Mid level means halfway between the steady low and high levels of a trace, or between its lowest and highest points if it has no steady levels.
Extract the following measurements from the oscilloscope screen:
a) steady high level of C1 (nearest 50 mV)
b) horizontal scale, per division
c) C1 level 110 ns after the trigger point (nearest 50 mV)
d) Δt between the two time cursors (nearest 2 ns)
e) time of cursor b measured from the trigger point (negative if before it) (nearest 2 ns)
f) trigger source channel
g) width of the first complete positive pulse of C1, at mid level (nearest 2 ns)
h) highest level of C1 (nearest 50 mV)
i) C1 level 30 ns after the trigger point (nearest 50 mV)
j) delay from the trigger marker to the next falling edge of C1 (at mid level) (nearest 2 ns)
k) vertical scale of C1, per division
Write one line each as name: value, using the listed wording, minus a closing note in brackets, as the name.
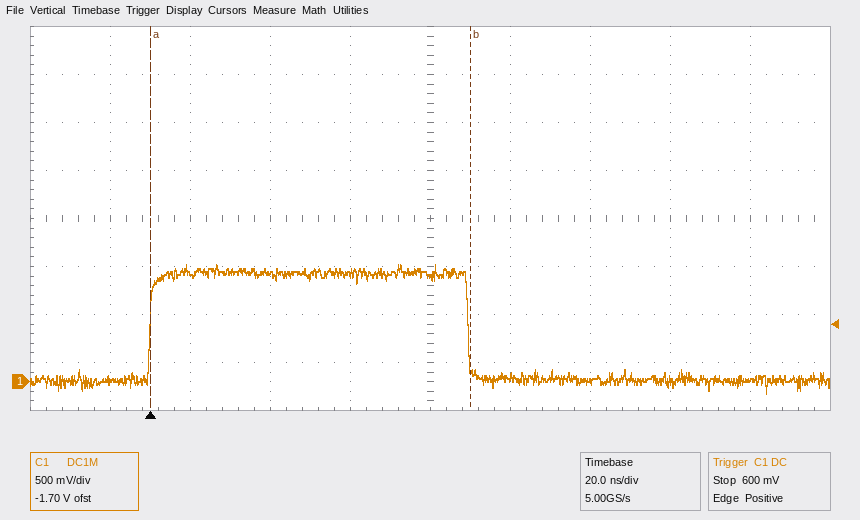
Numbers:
steady high level of C1: 1.15 V
horizontal scale, per division: 20 ns
C1 level 110 ns after the trigger point: 0 mV
Δt between the two time cursors: 80 ns
time of cursor b measured from the trigger point (negative if before it): +80 ns
trigger source channel: C1
width of the first complete positive pulse of C1, at mid level: 80 ns
highest level of C1: 1.20 V
C1 level 30 ns after the trigger point: 1.10 V
delay from the trigger marker to the next falling edge of C1 (at mid level): 80 ns
vertical scale of C1, per division: 500 mV
